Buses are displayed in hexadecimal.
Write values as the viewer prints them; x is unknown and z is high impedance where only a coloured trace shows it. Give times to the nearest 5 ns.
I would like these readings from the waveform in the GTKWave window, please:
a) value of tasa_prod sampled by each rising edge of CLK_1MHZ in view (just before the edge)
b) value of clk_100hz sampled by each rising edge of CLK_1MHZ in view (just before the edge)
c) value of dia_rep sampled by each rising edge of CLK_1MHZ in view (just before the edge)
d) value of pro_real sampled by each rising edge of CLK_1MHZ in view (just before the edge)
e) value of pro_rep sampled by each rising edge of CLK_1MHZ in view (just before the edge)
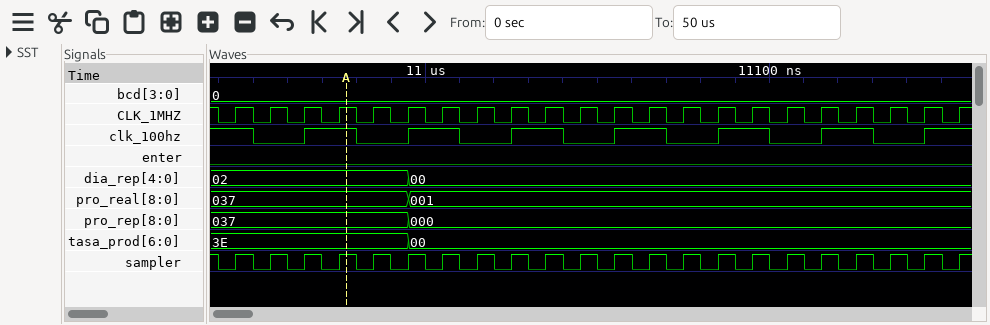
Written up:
3E, 3E, 3E, 3E, 3E, 3E, 00, 00, 00, 00, 00, 00, 00, 00, 00, 00, 00, 00, 00, 00, 00, 00
1 0 0 1 0 0 1 0 0 1 0 0 1 0 0 1 0 0 1 0 0 1
02, 02, 02, 02, 02, 02, 00, 00, 00, 00, 00, 00, 00, 00, 00, 00, 00, 00, 00, 00, 00, 00
037, 037, 037, 037, 037, 037, 001, 001, 001, 001, 001, 001, 001, 001, 001, 001, 001, 001, 001, 001, 001, 001
037, 037, 037, 037, 037, 037, 000, 000, 000, 000, 000, 000, 000, 000, 000, 000, 000, 000, 000, 000, 000, 000
